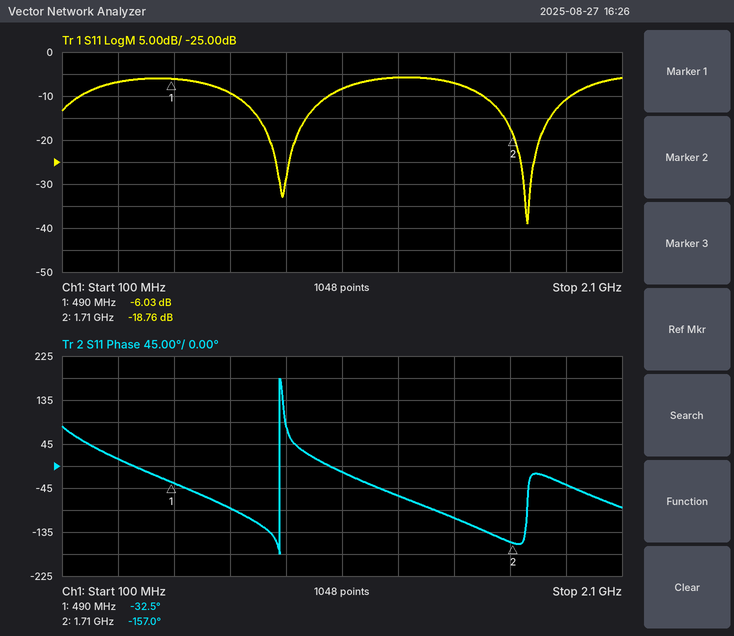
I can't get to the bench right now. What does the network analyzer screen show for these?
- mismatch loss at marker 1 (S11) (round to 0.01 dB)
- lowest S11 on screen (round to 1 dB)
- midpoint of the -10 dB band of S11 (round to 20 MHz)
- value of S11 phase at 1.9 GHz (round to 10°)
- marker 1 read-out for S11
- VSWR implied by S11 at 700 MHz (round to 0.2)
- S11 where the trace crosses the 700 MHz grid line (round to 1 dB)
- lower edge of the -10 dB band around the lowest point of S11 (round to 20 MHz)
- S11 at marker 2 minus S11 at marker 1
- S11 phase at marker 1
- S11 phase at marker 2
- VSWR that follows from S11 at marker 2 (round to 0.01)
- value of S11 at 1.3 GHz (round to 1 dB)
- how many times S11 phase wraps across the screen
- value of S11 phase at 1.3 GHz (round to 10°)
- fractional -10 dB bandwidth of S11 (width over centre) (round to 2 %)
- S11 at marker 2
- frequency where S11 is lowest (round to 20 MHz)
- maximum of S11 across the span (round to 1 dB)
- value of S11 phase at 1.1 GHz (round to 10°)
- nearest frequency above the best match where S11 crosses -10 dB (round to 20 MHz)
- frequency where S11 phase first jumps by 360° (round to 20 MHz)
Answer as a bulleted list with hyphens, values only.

- 1.25 dB
- -39 dB
- 1.76 GHz
- -40°
- -6.03 dB
- 2.0
- -9 dB
- 1.60 GHz
- -12.73 dB
- -32.5°
- -157.0°
- 1.26
- -6 dB
- 1
- -60°
- 18 %
- -18.76 dB
- 1.76 GHz
- -6 dB
- -10°
- 1.92 GHz
- 880 MHz
